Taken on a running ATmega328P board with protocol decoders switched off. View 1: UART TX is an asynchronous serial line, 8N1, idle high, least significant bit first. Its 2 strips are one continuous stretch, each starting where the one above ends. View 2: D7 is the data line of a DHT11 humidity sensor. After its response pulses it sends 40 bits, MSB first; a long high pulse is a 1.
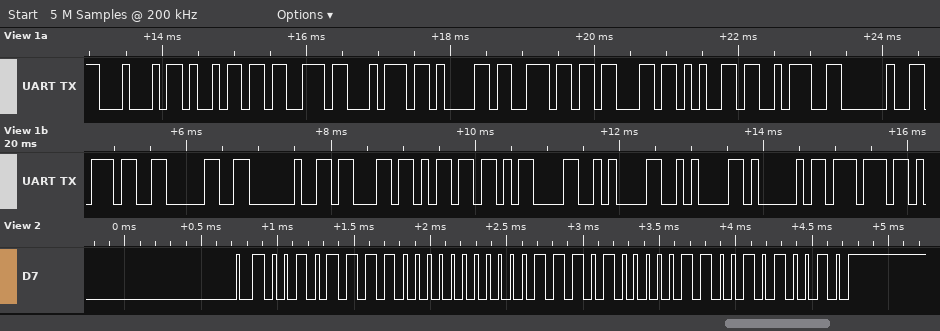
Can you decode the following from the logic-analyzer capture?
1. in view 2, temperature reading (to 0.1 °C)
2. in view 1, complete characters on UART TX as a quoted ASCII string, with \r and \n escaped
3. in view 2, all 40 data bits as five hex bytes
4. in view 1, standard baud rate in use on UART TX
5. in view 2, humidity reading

29.6 °C
"Distance: 70 cm\r\n\nAw"
2F 00 1D 06 52
9600 baud
47 %
